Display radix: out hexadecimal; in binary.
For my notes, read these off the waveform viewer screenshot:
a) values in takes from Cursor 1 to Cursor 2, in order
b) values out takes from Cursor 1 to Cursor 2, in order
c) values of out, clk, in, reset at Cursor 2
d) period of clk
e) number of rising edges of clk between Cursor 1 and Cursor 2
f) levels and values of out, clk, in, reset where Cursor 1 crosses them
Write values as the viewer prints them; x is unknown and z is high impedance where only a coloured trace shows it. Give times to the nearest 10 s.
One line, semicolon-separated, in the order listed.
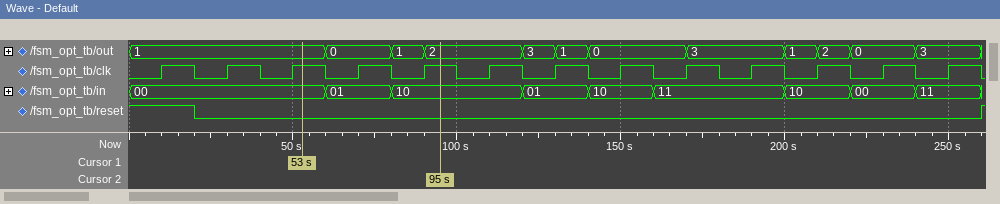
00, 01, 10; 1, 0, 1, 2; out=2, clk=1, in=10, reset=0; 20 s; 2; out=1, clk=1, in=00, reset=0
